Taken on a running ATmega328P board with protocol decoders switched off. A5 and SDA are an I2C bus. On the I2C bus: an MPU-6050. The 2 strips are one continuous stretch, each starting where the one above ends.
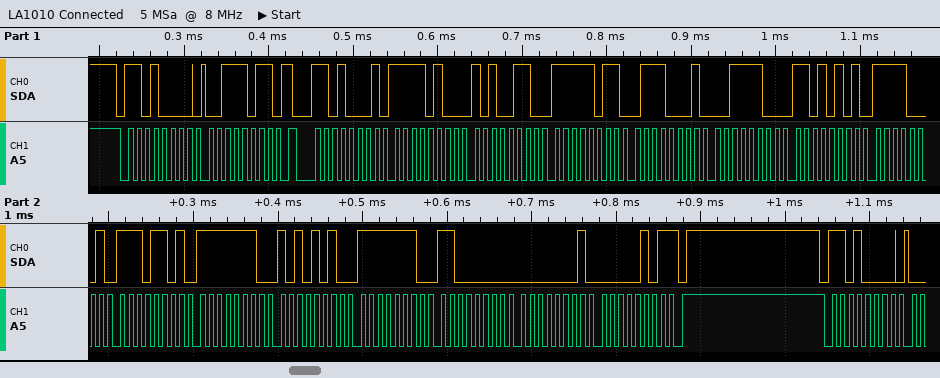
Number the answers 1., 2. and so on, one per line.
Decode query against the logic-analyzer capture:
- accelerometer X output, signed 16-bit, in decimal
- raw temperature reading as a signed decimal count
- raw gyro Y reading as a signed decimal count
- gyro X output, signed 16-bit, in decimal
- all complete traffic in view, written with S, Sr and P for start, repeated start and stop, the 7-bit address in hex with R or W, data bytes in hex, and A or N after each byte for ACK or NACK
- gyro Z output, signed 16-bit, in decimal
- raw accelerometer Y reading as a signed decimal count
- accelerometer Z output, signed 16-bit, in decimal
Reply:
1. -2906
2. -3603
3. -320
4. -342
5. S 68W A 3B A Sr 68R A F4 A A6 A FB A 71 A 3C A D5 A F1 A ED A FE A AA A FE A C0 A 01 A 05 N P S 68W A
6. 261
7. -1167
8. 15573
